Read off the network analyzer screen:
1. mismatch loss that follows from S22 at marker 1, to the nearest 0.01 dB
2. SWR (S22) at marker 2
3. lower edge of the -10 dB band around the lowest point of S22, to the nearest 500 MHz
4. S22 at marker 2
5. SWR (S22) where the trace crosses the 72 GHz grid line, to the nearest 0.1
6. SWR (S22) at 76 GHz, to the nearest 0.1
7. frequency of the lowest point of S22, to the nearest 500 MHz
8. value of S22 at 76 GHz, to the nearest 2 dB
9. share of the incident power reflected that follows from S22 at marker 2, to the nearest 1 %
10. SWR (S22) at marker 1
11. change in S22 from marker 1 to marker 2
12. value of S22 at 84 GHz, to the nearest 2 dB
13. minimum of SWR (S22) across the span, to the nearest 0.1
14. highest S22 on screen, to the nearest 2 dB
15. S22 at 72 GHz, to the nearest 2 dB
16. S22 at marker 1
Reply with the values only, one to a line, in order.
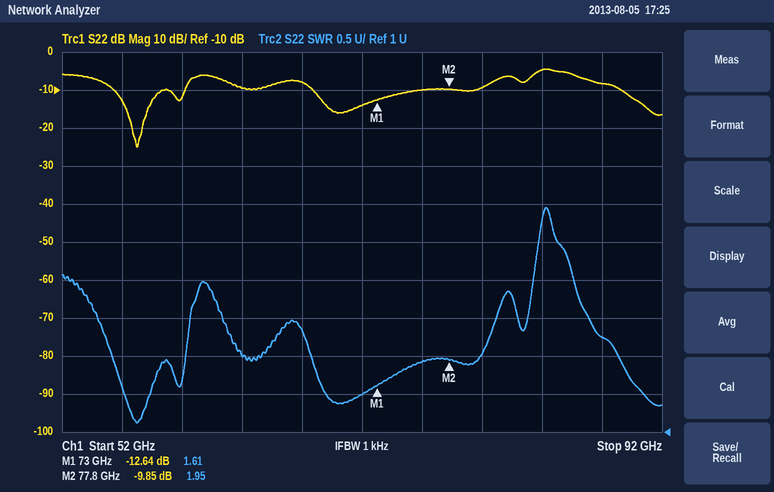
0.24 dB
1.95
55.5 GHz
-9.85 dB
1.5
1.9
57.0 GHz
-10 dB
10 %
1.61
2.79 dB
-4 dB
1.1
-4 dB
-14 dB
-12.64 dB
